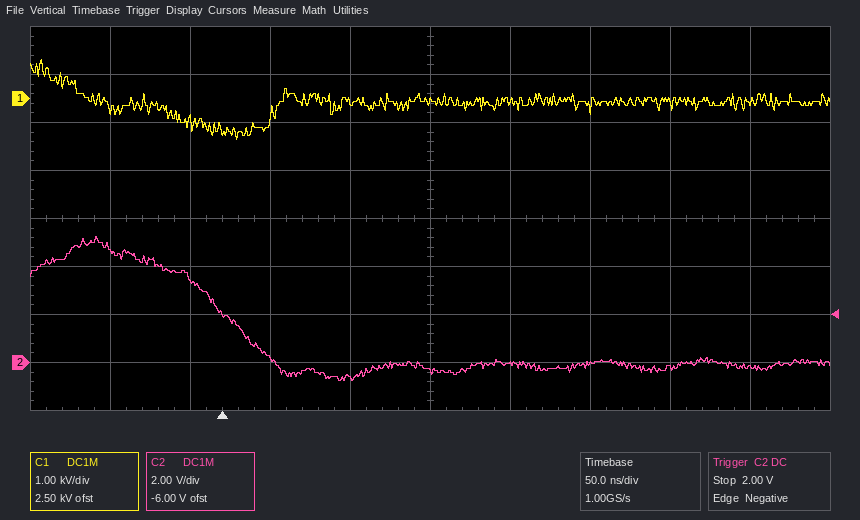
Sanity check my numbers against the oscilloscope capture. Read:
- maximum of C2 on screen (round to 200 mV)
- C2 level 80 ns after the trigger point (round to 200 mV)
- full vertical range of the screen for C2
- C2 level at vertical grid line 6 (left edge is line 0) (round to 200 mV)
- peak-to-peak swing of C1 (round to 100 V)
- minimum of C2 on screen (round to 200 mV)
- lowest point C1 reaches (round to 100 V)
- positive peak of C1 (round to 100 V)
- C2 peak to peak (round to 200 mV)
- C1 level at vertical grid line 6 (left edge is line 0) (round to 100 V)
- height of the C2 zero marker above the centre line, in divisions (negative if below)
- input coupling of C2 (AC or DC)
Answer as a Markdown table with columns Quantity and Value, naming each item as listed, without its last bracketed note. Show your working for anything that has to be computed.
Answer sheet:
| Quantity | Value |
|---|---|
| maximum of C2 on screen | 5.2 V |
| C2 level 80 ns after the trigger point | -600 mV |
| full vertical range of the screen for C2 | 16 V |
| C2 level at vertical grid line 6 (left edge is line 0) | 0.0 V |
| peak-to-peak swing of C1 | 800 V − (-900 V) = 1.7 kV |
| minimum of C2 on screen | -800 mV |
| lowest point C1 reaches | -900 V |
| positive peak of C1 | 800 V |
| C2 peak to peak | 5.2 V − (-800 mV) = 6.0 V |
| C1 level at vertical grid line 6 (left edge is line 0) | -100 V |
| height of the C2 zero marker above the centre line, in divisions | -3.0 div |
| input coupling of C2 | DC |
